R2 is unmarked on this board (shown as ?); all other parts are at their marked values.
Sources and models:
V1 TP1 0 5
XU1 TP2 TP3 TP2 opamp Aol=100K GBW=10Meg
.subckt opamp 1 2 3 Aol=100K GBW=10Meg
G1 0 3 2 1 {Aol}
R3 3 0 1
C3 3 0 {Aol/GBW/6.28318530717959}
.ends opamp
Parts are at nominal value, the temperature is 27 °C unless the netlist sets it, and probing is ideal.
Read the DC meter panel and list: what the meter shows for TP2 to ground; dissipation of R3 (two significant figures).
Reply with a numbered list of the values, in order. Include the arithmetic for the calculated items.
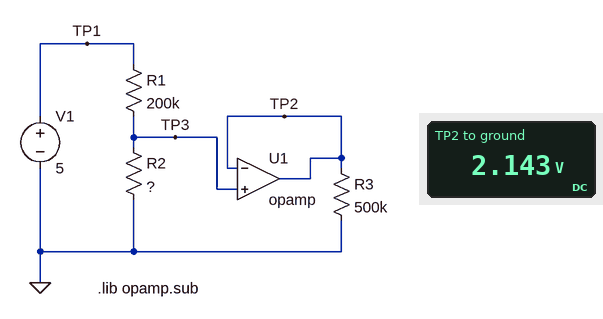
1. 2.143 V
2. (2.143 V)^2 / 500 kΩ = 9.2 µW
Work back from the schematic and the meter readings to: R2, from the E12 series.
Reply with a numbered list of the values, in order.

1. 150 kΩ
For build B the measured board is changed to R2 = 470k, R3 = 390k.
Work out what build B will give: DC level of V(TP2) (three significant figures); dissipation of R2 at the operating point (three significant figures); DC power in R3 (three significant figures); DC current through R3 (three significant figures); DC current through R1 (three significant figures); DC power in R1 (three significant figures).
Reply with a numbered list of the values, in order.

1. 3.51 V
2. 26.2 µW
3. 31.5 µW
4. 8.99 µA
5. 7.46 µA
6. 11.1 µW
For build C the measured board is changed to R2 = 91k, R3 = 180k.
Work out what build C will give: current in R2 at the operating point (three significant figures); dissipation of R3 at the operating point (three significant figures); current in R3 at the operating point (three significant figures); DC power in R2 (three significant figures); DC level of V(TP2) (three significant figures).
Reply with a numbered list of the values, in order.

1. 17.2 µA
2. 13.6 µW
3. 8.69 µA
4. 26.9 µW
5. 1.56 V
